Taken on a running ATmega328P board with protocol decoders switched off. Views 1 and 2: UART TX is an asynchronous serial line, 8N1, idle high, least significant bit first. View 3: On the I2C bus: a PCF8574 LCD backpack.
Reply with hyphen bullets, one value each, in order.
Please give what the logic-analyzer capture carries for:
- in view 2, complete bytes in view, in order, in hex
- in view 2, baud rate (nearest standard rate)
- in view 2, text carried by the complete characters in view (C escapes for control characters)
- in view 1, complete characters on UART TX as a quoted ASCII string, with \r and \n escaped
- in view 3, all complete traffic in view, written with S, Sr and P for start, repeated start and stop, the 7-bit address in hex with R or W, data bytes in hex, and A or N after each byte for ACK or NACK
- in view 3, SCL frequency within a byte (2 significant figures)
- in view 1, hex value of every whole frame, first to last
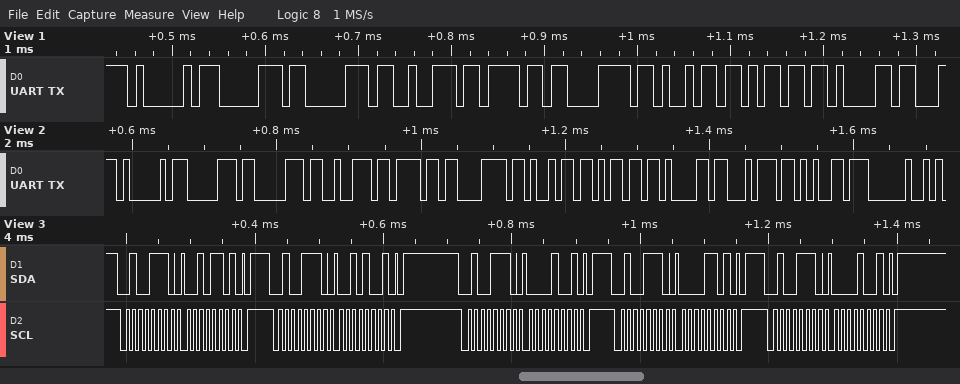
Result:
- 41 70 70 72 6F 78 69 6D 61 74 65 20
- 115200 baud
- "Approximate "
- "Approxima"
- S 27W A 2D A P S 27W A 29 A P S 27W A 09 A P S 27W A 0D A P S 27W A 09 A P
- 100 kHz
- 0x41 0x70 0x70 0x72 0x6F 0x78 0x69 0x6D 0x61
